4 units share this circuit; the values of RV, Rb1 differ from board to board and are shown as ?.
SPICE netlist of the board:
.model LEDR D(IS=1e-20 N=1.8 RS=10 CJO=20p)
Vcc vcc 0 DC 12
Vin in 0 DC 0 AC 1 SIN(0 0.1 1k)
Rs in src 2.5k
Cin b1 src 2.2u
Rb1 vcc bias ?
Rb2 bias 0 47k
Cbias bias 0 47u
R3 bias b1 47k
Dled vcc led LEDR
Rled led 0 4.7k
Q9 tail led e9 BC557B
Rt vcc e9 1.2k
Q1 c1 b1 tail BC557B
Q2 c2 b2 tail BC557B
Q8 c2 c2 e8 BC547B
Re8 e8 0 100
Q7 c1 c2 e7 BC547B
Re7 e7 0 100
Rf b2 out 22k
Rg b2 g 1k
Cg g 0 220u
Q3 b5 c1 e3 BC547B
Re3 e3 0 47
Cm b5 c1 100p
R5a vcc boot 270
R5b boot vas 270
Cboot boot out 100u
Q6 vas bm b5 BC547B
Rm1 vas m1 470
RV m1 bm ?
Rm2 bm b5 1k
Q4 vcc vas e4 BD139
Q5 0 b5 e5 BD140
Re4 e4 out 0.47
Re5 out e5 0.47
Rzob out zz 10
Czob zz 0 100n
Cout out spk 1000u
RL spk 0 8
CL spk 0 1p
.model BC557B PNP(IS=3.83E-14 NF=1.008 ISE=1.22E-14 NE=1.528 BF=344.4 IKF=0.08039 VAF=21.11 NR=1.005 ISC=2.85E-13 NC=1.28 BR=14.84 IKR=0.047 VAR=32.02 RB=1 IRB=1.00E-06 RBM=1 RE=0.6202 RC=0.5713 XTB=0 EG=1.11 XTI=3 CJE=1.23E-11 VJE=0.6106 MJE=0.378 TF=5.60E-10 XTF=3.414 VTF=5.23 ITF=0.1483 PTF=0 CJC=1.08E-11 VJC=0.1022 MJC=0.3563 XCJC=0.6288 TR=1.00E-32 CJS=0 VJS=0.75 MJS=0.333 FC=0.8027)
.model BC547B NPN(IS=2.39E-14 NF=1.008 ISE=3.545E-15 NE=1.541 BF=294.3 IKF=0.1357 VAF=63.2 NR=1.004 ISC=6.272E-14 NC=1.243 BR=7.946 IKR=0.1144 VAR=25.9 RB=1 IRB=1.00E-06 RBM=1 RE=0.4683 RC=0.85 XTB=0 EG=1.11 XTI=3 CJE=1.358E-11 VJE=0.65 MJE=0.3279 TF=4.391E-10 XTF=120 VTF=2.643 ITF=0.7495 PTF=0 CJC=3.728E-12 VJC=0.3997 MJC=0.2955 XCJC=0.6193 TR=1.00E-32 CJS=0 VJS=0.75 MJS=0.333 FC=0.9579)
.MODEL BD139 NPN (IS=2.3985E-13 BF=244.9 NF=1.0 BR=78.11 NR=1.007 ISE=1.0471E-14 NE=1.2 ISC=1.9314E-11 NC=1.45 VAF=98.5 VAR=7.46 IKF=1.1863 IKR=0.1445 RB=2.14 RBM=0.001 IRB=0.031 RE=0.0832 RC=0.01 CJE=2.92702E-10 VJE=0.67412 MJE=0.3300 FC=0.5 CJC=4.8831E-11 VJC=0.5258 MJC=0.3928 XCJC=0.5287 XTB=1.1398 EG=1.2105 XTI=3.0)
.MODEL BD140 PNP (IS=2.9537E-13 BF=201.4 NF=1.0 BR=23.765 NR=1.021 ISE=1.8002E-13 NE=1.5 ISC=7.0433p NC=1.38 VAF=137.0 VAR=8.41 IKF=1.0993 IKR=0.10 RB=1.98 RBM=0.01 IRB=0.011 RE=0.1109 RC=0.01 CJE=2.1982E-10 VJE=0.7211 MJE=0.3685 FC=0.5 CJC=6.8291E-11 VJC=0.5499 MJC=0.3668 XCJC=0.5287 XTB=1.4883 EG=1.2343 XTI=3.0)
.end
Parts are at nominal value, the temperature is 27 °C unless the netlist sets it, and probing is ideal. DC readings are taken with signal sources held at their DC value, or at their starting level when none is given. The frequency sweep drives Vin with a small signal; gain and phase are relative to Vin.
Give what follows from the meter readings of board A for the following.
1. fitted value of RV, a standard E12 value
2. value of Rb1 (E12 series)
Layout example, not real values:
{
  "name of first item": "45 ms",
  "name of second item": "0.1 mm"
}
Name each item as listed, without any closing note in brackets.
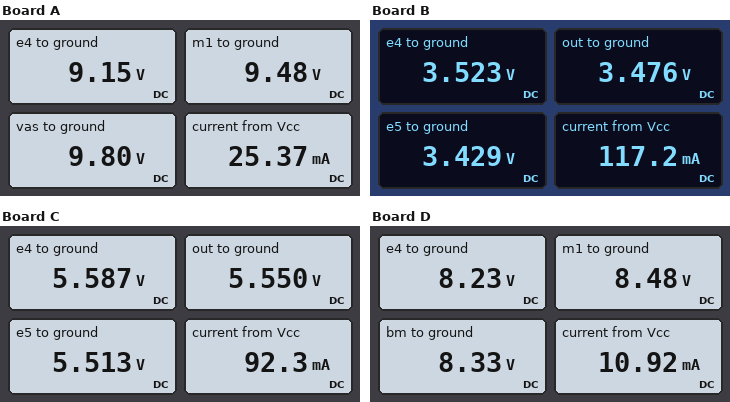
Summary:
{
  "fitted value of RV, a standard E12 value": "470 Ω",
  "value of Rb1": "15 kΩ"
}
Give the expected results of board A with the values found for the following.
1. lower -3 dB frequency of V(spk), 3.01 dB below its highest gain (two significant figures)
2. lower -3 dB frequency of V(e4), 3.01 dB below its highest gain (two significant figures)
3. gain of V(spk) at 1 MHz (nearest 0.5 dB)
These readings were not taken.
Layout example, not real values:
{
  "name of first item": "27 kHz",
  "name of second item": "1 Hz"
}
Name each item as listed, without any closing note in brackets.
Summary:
{
  "lower -3 dB frequency of V(spk), 3.01 dB below its highest gain": "21 Hz",
  "lower -3 dB frequency of V(e4), 3.01 dB below its highest gain": "2.1 Hz",
  "gain of V(spk) at 1 MHz": "25.5 dB"
}
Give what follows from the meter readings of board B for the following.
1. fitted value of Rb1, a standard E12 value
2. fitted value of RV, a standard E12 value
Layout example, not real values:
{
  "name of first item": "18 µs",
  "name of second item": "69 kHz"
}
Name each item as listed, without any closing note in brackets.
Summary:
{
  "fitted value of Rb1, a standard E12 value": "120 kΩ",
  "fitted value of RV, a standard E12 value": "560 Ω"
}
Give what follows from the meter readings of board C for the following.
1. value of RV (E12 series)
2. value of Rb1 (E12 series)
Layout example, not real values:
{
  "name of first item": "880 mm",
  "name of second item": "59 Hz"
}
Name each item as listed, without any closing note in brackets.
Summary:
{
  "value of RV": "560 Ω",
  "value of Rb1": "56 kΩ"
}
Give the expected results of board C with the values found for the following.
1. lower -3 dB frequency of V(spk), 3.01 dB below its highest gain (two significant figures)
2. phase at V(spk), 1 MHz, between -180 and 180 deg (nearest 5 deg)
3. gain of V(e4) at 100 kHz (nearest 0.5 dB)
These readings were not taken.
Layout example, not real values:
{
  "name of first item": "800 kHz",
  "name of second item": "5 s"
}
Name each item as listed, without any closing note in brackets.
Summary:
{
  "lower -3 dB frequency of V(spk), 3.01 dB below its highest gain": "20 Hz",
  "phase at V(spk), 1 MHz, between -180 and 180 deg": "-70 deg",
  "gain of V(e4) at 100 kHz": "27.0 dB"
}
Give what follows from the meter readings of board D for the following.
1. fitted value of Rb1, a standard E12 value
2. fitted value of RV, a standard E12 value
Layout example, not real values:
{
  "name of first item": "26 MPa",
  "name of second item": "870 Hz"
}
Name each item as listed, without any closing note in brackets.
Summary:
{
  "fitted value of Rb1, a standard E12 value": "22 kΩ",
  "fitted value of RV, a standard E12 value": "220 Ω"
}
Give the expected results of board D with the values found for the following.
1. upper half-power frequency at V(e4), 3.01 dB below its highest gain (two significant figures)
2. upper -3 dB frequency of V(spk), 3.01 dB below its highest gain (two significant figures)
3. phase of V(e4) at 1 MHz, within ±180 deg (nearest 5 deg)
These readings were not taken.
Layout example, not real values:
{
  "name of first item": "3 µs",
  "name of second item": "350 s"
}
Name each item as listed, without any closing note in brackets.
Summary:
{
  "upper half-power frequency at V(e4), 3.01 dB below its highest gain": "480 kHz",
  "upper -3 dB frequency of V(spk), 3.01 dB below its highest gain": "470 kHz",
  "phase of V(e4) at 1 MHz, within ±180 deg": "-120 deg"
}
